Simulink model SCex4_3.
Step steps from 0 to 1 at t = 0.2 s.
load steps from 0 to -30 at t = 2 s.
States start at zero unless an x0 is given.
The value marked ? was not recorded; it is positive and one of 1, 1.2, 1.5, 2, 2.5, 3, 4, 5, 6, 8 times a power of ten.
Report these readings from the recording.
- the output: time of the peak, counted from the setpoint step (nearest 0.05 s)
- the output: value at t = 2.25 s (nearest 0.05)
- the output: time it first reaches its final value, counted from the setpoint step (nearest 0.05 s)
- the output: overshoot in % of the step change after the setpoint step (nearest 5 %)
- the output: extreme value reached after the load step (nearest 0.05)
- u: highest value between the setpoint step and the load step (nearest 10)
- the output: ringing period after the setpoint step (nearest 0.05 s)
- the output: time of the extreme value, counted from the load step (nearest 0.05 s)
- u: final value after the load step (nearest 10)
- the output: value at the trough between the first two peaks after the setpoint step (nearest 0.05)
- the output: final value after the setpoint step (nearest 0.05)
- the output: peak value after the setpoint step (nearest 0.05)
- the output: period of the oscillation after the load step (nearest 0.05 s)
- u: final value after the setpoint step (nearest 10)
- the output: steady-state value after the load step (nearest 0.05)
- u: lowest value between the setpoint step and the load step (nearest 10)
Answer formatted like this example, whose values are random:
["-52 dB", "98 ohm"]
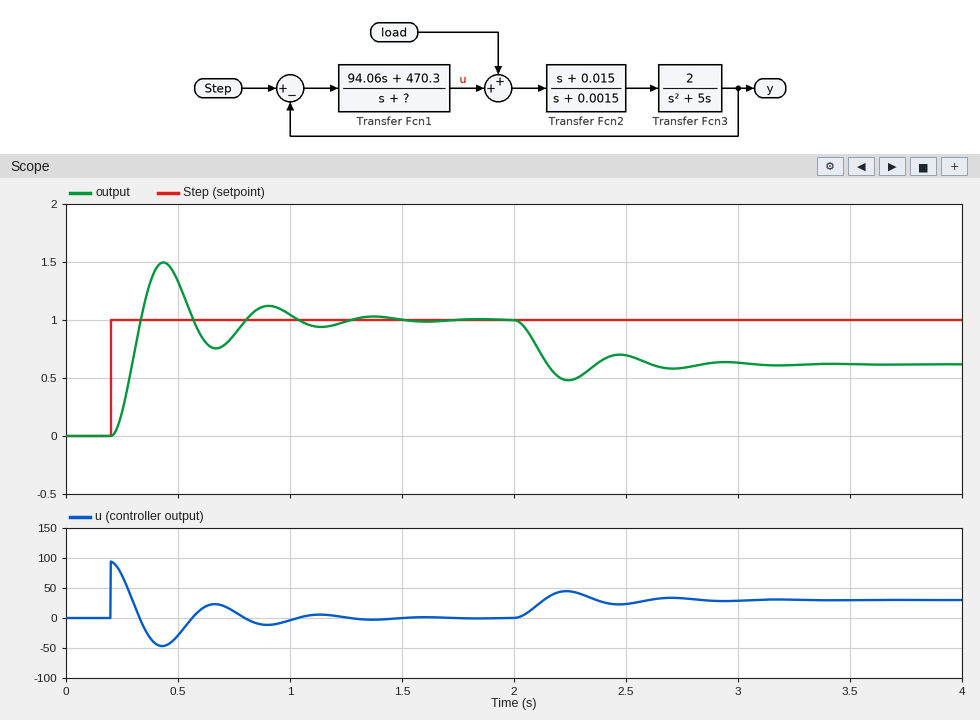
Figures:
["0.25 s", "0.50", "0.15 s", "50 %", "0.50", "90", "0.45 s", "0.25 s", "30", "0.75", "1.00", "1.50", "0.45 s", "0", "0.60", "-50"]
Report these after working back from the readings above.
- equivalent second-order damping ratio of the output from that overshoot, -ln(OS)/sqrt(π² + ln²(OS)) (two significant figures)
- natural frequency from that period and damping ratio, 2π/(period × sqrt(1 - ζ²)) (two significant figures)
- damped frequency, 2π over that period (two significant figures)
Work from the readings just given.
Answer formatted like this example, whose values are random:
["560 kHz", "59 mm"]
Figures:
["0.22", "14 rad/s", "14 rad/s"]
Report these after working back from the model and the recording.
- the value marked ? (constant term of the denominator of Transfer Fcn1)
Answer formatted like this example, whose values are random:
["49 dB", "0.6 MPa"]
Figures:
["6"]
